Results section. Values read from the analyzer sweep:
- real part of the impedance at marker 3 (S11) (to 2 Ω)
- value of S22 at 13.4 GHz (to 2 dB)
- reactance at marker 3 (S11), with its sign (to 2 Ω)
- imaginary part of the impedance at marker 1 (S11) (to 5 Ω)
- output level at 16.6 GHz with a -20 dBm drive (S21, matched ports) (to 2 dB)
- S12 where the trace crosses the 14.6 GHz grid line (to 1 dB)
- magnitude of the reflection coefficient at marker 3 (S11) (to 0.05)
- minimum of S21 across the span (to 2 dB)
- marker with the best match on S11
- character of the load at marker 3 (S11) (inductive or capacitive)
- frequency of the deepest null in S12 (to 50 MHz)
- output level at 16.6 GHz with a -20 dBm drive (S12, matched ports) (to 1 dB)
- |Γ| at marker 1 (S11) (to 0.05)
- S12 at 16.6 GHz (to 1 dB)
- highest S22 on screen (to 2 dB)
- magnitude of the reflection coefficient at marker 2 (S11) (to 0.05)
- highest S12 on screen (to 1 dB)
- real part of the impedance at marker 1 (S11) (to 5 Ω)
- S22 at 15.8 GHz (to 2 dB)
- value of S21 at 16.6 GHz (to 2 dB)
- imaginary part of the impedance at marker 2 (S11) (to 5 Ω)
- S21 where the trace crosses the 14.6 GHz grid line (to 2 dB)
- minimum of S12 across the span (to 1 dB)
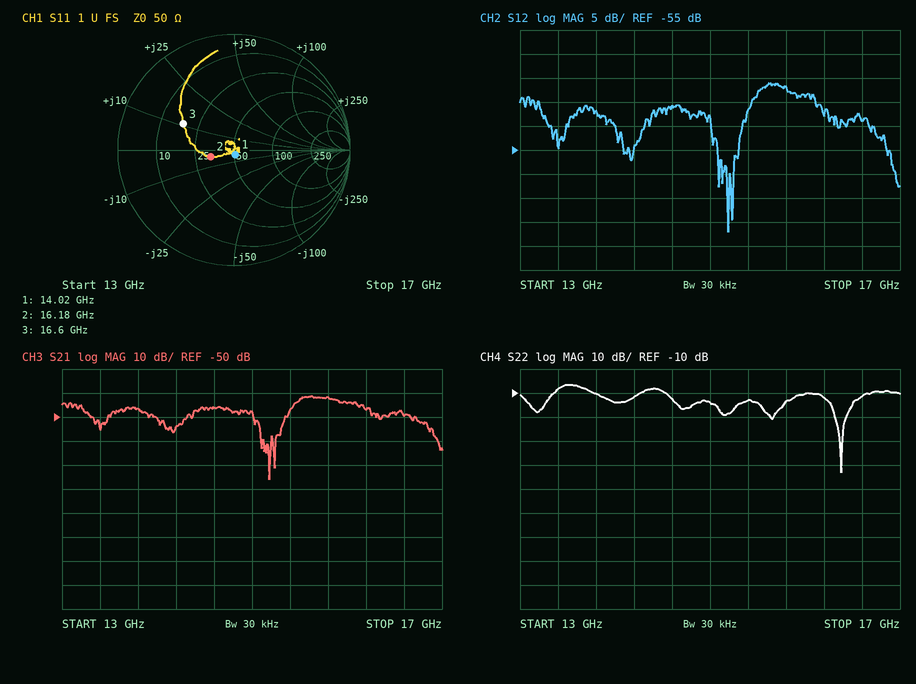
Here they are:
18 Ω
-8 dB
+10 Ω
-5 Ω
-70 dBm
-46 dB
0.50
-76 dB
marker 1
inductive
15.20 GHz
-69 dBm
0.05
-49 dB
-6 dB
0.20
-41 dB
50 Ω
-14 dB
-50 dB
-5 Ω
-46 dB
-72 dB
